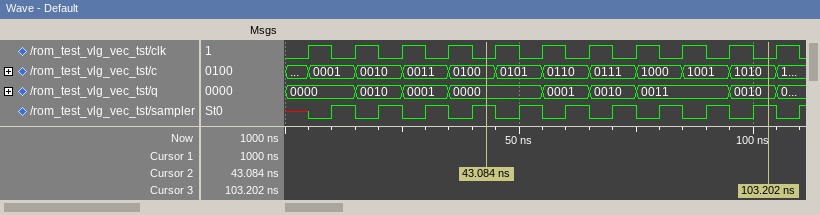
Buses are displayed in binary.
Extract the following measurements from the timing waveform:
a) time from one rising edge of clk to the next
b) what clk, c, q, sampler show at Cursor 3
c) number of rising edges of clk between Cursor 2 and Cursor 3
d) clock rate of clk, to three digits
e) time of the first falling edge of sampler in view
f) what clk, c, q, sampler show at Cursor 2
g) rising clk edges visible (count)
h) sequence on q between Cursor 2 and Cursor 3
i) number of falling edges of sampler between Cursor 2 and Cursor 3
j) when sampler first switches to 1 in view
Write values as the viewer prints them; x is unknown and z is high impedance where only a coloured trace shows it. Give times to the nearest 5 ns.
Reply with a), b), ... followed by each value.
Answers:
a) 10 ns
b) clk=0, c=1010, q=0010, sampler=1
c) 6
d) 100 MHz
e) 15 ns
f) clk=0, c=0100, q=0000, sampler=1
g) 11
h) 0000, 0001, 0010, 0011, 0010
i) 6
j) 10 ns
